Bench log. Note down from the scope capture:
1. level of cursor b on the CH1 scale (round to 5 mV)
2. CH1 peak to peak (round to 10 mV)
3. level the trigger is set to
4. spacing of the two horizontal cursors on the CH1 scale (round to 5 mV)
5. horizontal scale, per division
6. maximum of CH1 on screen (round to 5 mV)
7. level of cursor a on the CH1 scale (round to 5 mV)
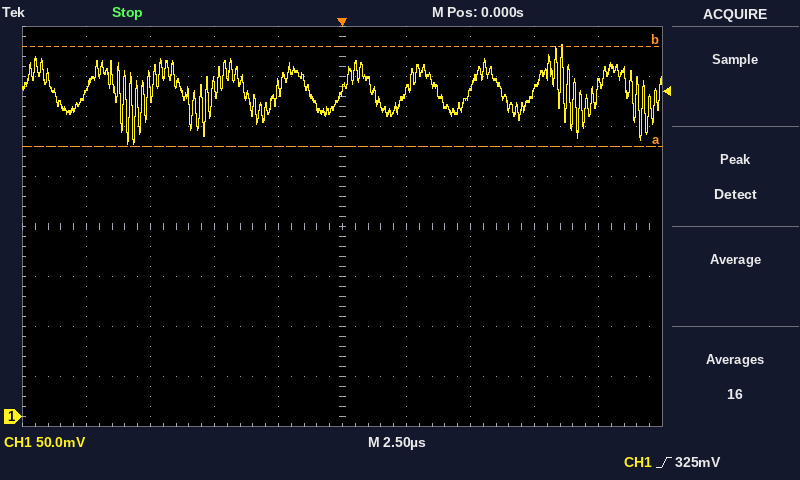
370 mV
100 mV
325 mV
100 mV
2.5 µs
370 mV
270 mV
